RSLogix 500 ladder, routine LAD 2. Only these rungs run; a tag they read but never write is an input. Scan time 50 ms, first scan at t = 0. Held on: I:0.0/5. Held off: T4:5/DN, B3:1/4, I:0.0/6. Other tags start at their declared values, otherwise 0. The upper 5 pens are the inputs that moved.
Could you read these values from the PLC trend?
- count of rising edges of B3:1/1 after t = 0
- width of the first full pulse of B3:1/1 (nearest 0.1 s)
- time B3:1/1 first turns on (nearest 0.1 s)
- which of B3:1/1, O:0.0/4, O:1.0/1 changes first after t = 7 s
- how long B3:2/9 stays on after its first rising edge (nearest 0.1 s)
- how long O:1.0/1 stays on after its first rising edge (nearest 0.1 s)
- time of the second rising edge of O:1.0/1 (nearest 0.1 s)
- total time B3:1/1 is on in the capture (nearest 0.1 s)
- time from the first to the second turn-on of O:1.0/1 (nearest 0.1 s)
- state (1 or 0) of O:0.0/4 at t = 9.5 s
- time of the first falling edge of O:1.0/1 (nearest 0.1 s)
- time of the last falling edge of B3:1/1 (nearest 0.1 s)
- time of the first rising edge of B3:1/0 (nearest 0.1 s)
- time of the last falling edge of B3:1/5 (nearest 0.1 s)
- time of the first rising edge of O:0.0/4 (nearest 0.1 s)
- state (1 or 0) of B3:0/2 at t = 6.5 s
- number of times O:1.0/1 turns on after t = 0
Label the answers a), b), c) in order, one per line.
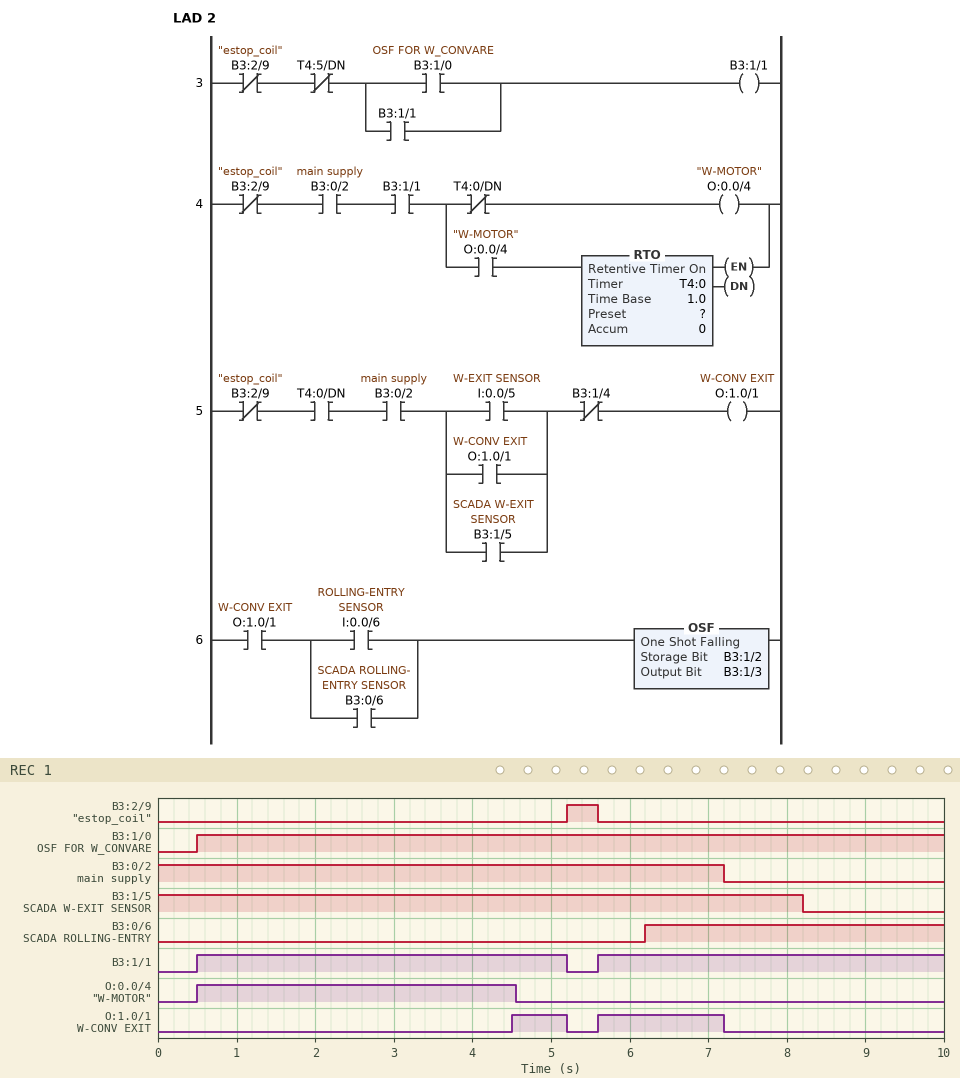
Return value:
a) 2
b) 4.7 s
c) 0.5 s
d) O:1.0/1
e) 0.4 s
f) 0.7 s
g) 5.6 s
h) 9.1 s
i) 1.1 s
j) 0
k) 5.2 s
l) 5.2 s
m) 0.5 s
n) 8.2 s
o) 0.5 s
p) 1
q) 2
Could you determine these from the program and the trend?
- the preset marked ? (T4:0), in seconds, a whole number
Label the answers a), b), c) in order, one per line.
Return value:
a) 4 s
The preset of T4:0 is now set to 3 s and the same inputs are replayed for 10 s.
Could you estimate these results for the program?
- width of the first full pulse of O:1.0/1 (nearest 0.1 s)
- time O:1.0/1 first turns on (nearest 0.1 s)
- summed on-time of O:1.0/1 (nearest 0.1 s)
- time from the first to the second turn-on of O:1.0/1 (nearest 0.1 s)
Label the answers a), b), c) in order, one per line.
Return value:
a) 1.7 s
b) 3.5 s
c) 3.3 s
d) 2.1 s
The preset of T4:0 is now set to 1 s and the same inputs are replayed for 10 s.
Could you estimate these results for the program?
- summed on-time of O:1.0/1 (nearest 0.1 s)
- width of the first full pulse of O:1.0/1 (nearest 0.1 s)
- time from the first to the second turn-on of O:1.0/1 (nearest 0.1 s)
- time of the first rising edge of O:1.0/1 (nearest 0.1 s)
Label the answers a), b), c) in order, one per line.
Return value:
a) 5.3 s
b) 3.7 s
c) 4.1 s
d) 1.5 s
